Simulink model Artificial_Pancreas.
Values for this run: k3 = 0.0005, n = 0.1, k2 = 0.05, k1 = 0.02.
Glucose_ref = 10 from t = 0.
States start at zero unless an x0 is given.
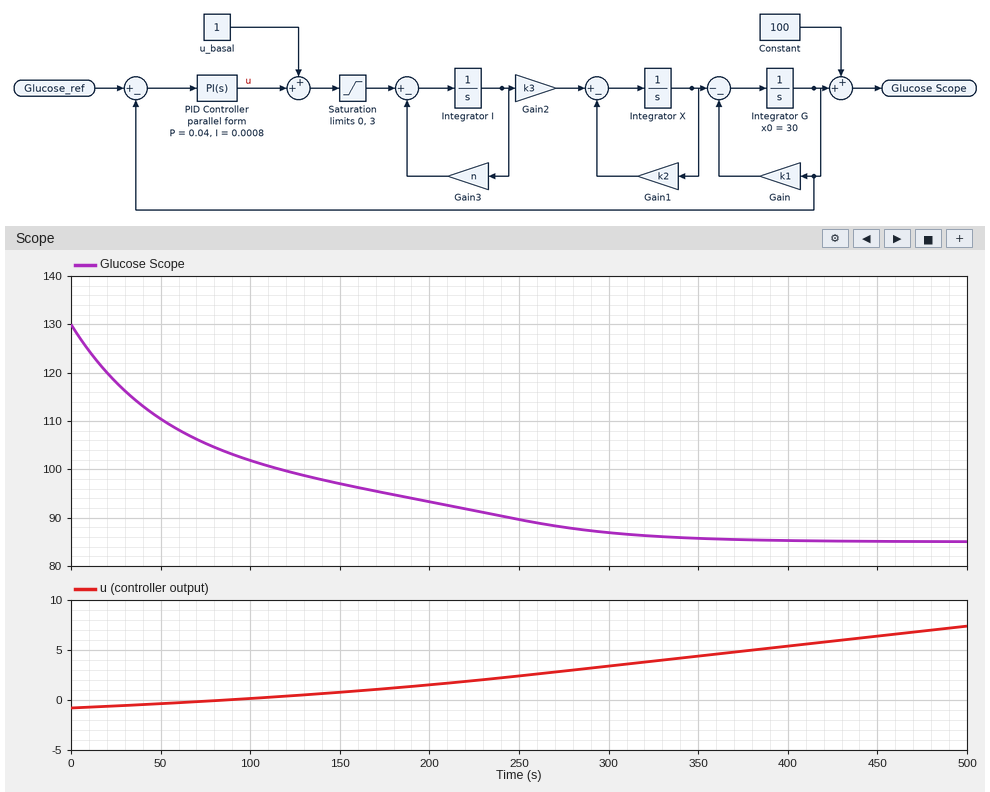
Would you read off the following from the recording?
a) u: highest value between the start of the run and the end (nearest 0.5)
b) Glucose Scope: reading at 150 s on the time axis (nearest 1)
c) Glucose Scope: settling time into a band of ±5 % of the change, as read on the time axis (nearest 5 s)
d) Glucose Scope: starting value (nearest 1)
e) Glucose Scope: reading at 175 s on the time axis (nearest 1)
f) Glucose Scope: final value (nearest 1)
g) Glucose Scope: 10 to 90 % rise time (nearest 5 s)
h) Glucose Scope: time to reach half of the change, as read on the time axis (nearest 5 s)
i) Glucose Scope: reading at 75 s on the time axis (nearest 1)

7.5
97
290 s
130
95
85
245 s
65 s
105
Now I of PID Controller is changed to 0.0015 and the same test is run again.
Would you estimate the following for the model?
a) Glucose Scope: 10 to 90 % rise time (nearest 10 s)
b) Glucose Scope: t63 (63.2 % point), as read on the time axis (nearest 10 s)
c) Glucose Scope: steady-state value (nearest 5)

230 s
110 s
85
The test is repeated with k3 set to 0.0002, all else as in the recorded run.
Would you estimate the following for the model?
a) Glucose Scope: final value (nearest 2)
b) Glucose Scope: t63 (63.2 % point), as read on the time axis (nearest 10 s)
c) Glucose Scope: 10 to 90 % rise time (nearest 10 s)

94
70 s
210 s
